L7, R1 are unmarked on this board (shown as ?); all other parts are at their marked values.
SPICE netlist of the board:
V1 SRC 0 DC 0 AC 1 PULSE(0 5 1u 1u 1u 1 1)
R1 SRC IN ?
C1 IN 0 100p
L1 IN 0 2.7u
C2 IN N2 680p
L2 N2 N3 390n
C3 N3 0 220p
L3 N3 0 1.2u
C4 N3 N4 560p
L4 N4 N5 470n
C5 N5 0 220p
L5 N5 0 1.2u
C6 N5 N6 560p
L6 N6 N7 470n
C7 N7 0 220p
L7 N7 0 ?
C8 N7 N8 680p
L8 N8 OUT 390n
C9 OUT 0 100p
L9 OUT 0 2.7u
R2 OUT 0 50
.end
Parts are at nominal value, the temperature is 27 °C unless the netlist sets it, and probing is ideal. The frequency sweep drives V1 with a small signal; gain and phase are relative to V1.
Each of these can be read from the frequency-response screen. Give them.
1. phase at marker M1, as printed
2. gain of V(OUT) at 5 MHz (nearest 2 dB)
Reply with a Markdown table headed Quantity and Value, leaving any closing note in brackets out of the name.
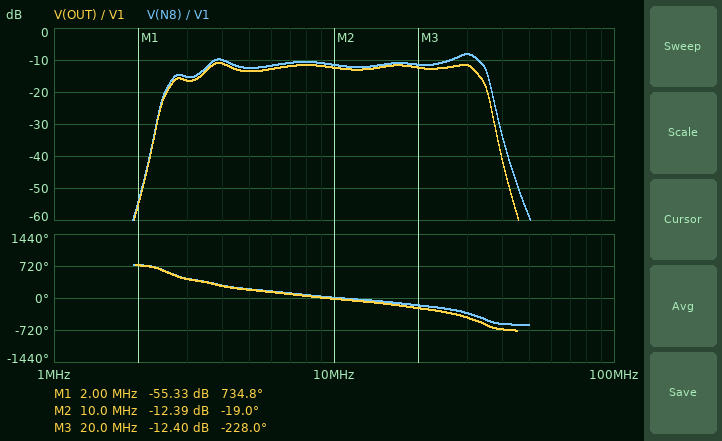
| Quantity | Value |
|---|---|
| phase at marker M1, as printed | 734.8 deg |
| gain of V(OUT) at 5 MHz | -14 dB |
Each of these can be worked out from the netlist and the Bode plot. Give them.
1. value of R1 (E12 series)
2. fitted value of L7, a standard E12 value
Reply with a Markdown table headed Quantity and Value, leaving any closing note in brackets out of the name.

| Quantity | Value |
|---|---|
| value of R1 | 150 Ω |
| fitted value of L7, a standard E12 value | 2.2 µH |
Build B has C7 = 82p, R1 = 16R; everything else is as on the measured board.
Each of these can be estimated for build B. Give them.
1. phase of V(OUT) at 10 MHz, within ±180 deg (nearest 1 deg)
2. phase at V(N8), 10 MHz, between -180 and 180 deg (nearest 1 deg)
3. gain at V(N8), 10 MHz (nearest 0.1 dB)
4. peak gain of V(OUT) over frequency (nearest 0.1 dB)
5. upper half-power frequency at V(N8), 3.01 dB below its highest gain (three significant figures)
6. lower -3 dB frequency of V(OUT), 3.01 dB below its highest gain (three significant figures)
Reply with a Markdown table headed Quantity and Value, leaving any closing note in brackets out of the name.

| Quantity | Value |
|---|---|
| phase of V(OUT) at 10 MHz, within ±180 deg | -4 deg |
| phase at V(N8), 10 MHz, between -180 and 180 deg | 23 deg |
| gain at V(N8), 10 MHz | -1.6 dB |
| peak gain of V(OUT) over frequency | -1.1 dB |
| upper half-power frequency at V(N8), 3.01 dB below its highest gain | 31.0 MHz |
| lower -3 dB frequency of V(OUT), 3.01 dB below its highest gain | 3.09 MHz |
